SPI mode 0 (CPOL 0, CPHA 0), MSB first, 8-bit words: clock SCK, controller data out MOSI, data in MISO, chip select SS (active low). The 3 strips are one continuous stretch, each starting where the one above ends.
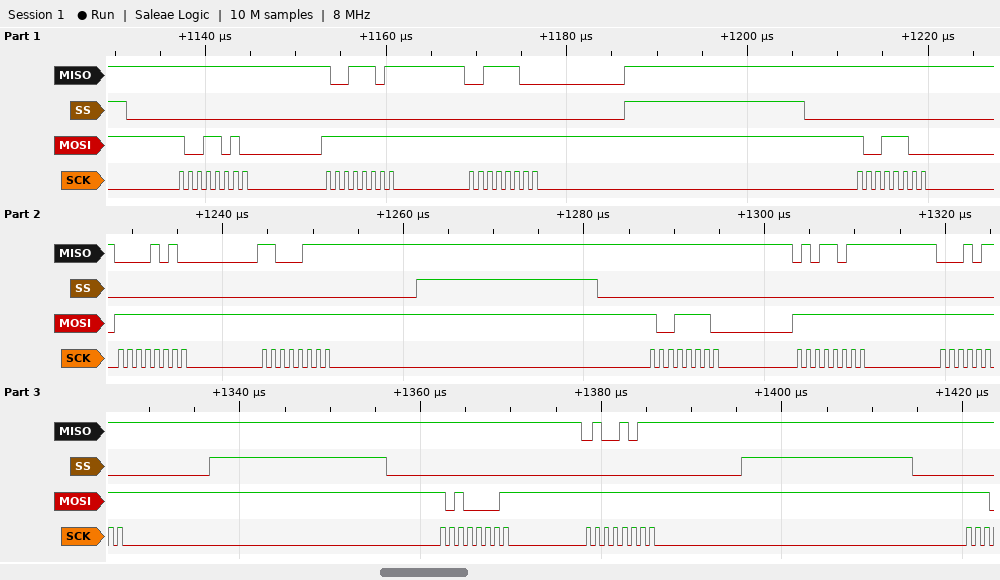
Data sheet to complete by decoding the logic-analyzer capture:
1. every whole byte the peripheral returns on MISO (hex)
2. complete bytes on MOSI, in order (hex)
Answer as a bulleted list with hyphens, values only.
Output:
- FF 9D 3C FF 0A C7 FF 5B 17 FF 4B
- 9A FF FF 9C FF FF 9E FF FF A1 FF
